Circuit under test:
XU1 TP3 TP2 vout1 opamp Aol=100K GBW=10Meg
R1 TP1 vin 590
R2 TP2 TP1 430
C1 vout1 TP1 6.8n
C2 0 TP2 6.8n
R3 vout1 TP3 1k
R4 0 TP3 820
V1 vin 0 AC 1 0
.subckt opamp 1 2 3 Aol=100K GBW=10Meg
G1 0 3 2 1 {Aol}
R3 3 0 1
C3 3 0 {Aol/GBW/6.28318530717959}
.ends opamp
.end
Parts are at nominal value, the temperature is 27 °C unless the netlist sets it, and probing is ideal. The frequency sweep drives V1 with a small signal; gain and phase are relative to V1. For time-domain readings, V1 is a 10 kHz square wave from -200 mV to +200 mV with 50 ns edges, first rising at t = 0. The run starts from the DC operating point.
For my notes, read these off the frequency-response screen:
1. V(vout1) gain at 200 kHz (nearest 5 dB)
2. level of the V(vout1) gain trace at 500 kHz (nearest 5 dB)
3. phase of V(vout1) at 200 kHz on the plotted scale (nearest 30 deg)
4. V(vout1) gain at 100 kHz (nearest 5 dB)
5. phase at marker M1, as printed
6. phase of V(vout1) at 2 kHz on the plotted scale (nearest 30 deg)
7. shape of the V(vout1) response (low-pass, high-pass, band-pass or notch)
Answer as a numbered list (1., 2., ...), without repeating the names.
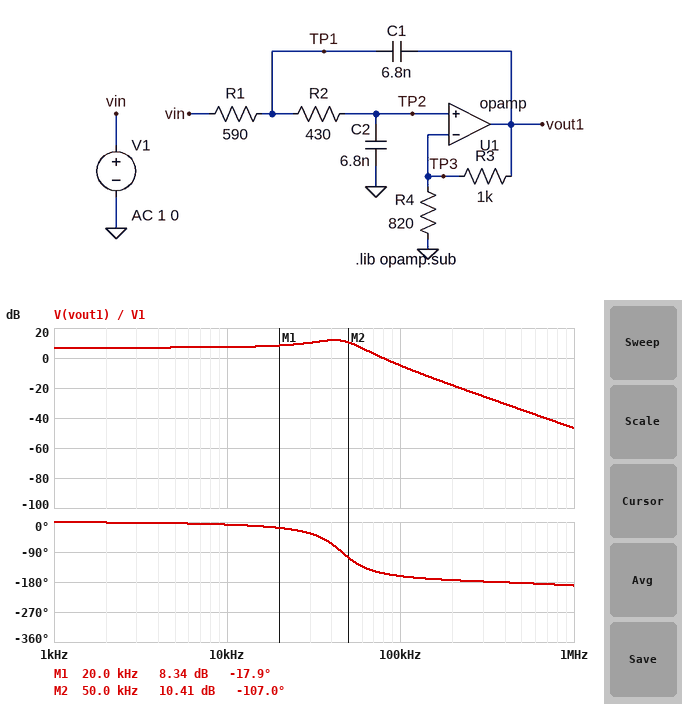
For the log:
1. -20 dB
2. -35 dB
3. -180 deg
4. -5 dB
5. -17.9 deg
6. 0 deg
7. low-pass
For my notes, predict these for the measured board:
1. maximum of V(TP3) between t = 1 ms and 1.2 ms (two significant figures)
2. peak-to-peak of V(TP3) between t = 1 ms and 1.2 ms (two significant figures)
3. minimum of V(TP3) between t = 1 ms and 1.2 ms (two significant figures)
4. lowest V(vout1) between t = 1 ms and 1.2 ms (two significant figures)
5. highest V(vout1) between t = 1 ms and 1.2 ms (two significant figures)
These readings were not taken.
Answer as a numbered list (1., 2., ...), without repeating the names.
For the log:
1. 350 mV
2. 700 mV
3. -350 mV
4. -780 mV
5. 780 mV
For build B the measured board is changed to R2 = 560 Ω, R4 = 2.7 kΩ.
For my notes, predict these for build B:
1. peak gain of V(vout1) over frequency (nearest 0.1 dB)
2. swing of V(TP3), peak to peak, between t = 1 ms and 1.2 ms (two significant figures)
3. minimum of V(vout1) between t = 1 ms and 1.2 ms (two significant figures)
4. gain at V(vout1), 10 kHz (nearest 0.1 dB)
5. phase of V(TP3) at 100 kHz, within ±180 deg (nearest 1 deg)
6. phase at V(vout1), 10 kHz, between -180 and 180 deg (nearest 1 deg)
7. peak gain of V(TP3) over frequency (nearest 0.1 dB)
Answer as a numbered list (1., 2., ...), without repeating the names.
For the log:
1. 2.7 dB
2. 410 mV
3. -280 mV
4. 2.6 dB
5. -143 deg
6. -23 deg
7. 0 dB
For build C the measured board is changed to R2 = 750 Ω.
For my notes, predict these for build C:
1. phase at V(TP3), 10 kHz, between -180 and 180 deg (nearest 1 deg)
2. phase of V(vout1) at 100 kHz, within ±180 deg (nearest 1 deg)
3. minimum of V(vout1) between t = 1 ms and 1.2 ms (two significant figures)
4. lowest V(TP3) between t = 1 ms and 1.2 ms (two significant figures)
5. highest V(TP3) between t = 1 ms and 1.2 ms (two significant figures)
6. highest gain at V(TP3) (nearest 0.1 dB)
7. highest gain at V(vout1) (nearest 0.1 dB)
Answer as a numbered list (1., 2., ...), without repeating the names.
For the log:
1. -16 deg
2. -161 deg
3. -620 mV
4. -280 mV
5. 280 mV
6. 1.7 dB
7. 8.6 dB
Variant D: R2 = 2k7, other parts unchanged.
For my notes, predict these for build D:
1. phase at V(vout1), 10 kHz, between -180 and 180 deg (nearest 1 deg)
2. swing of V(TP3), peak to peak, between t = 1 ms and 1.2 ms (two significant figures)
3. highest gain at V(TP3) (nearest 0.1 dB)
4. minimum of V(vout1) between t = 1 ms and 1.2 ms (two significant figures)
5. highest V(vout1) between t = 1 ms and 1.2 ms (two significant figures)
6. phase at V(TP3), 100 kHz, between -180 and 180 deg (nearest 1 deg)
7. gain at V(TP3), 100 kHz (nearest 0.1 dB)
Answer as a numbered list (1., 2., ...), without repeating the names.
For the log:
1. -57 deg
2. 380 mV
3. 0 dB
4. -420 mV
5. 420 mV
6. -160 deg
7. -29.6 dB
